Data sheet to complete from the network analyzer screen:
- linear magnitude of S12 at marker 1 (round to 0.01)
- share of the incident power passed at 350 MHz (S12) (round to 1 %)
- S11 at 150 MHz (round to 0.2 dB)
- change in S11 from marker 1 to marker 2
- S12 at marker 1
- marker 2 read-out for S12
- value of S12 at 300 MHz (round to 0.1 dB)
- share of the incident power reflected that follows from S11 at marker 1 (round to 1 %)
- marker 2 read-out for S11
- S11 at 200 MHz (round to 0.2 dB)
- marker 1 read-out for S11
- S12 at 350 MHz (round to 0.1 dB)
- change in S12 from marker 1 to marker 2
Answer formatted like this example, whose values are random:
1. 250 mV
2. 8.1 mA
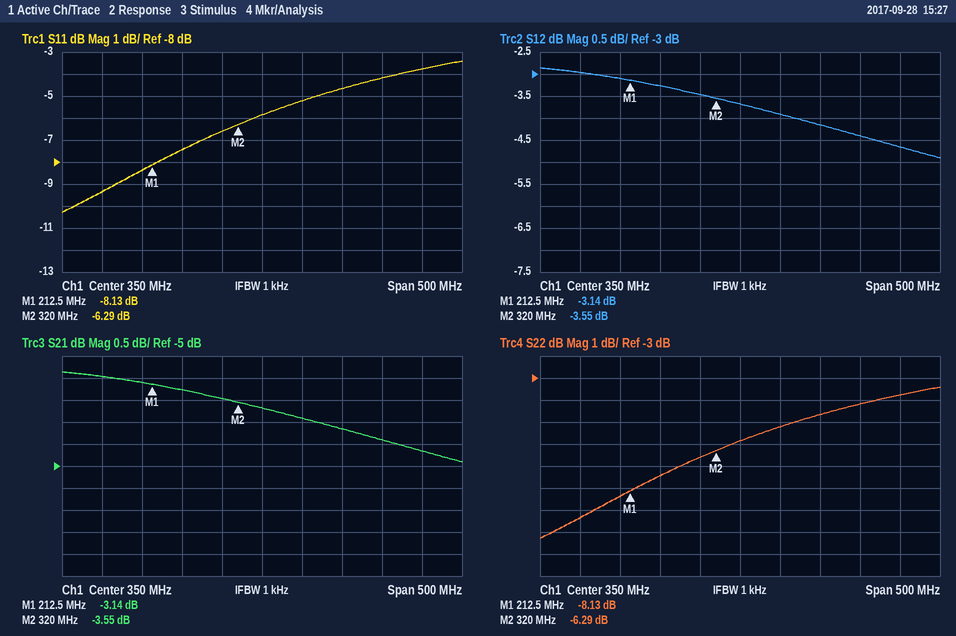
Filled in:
1. 0.70
2. 43 %
3. -9.4 dB
4. 1.84 dB
5. -3.14 dB
6. -3.55 dB
7. -3.5 dB
8. 15 %
9. -6.29 dB
10. -8.4 dB
11. -8.13 dB
12. -3.7 dB
13. -0.41 dB
